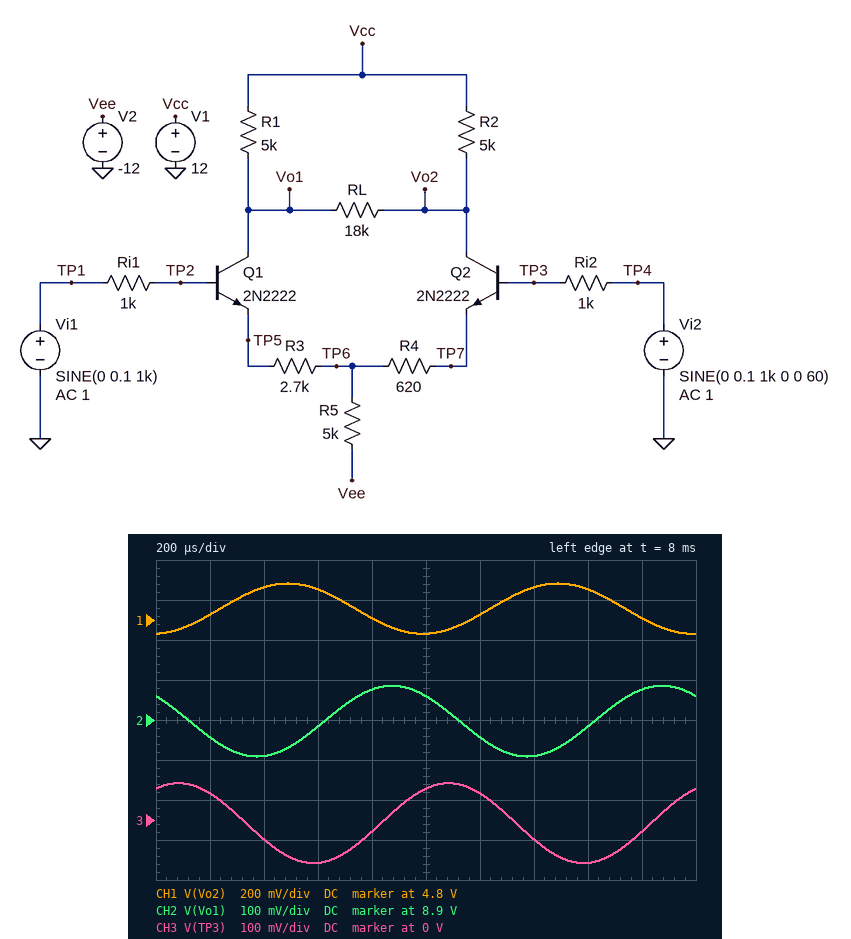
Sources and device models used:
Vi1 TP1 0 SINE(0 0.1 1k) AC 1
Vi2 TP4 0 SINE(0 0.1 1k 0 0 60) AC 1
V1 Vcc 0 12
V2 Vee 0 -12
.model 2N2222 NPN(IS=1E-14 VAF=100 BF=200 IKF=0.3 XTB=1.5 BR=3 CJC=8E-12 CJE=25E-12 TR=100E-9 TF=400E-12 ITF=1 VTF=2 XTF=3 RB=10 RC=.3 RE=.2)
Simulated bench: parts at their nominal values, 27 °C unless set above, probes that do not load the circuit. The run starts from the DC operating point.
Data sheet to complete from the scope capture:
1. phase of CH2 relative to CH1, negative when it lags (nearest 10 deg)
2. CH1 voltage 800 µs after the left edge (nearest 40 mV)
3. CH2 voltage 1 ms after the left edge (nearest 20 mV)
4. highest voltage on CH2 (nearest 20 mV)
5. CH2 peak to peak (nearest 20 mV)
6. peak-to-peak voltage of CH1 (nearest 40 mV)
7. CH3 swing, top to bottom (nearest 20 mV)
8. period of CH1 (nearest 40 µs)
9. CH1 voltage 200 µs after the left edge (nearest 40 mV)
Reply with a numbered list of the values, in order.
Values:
1. -140 deg
2. 4.80 V
3. 8.96 V
4. 8.98 V
5. 180 mV
6. 240 mV
7. 200 mV
8. 1.00 ms
9. 4.84 V
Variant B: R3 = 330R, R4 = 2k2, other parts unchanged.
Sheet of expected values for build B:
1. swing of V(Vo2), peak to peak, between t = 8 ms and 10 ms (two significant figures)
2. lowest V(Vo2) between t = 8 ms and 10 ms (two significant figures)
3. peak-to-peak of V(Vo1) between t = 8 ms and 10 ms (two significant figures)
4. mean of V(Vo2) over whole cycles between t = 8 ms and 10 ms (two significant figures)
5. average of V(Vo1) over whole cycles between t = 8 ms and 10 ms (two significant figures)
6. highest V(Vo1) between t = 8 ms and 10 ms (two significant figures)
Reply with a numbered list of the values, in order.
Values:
1. 230 mV
2. 9.0 V
3. 320 mV
4. 9.1 V
5. 4.2 V
6. 4.4 V
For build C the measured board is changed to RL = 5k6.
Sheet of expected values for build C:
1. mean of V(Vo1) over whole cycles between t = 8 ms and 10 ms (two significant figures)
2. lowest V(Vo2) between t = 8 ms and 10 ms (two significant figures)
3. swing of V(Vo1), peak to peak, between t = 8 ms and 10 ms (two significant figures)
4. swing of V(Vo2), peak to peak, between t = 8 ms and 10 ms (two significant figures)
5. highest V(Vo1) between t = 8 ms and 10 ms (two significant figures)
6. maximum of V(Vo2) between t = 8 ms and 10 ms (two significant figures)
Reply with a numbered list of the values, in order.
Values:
1. 8.0 V
2. 5.7 V
3. 100 mV
4. 170 mV
5. 8.1 V
6. 5.8 V
